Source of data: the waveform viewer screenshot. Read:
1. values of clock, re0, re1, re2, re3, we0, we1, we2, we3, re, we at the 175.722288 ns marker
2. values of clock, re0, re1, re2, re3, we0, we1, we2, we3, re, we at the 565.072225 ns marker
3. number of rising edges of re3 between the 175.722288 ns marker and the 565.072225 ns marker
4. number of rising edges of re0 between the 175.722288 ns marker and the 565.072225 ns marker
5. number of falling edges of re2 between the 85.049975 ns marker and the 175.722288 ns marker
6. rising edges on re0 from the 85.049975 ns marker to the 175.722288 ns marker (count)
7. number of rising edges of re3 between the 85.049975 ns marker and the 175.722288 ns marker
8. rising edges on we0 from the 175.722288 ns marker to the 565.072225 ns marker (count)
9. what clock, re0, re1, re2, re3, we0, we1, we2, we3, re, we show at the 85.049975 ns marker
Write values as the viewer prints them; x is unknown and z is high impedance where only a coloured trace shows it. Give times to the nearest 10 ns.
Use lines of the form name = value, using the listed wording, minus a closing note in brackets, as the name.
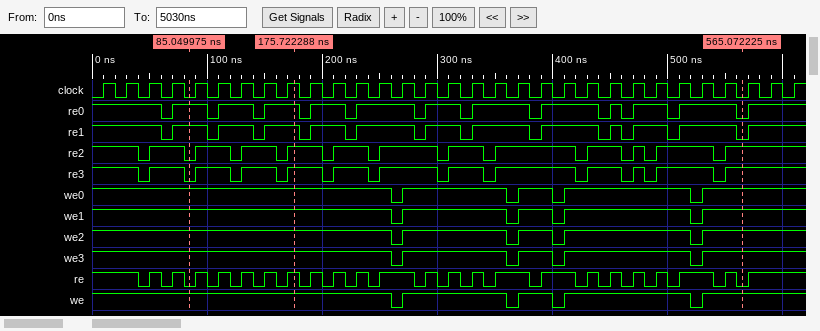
values of clock, re0, re1, re2, re3, we0, we1, we2, we3, re, we at the 175.722288 ns marker = clock=1, re0=1, re1=1, re2=1, re3=1, we0=1, we1=1, we2=1, we3=1, re=1, we=1
values of clock, re0, re1, re2, re3, we0, we1, we2, we3, re, we at the 565.072225 ns marker = clock=0, re0=0, re1=0, re2=1, re3=1, we0=1, we1=1, we2=1, we3=1, re=0, we=1
number of rising edges of re3 between the 175.722288 ns marker and the 565.072225 ns marker = 8
number of rising edges of re0 between the 175.722288 ns marker and the 565.072225 ns marker = 8
number of falling edges of re2 between the 85.049975 ns marker and the 175.722288 ns marker = 2
rising edges on re0 from the 85.049975 ns marker to the 175.722288 ns marker = 2
number of rising edges of re3 between the 85.049975 ns marker and the 175.722288 ns marker = 3
rising edges on we0 from the 175.722288 ns marker to the 565.072225 ns marker = 4
what clock, re0, re1, re2, re3, we0, we1, we2, we3, re, we show at the 85.049975 ns marker = clock=0, re0=1, re1=1, re2=0, re3=0, we0=1, we1=1, we2=1, we3=1, re=0, we=1
